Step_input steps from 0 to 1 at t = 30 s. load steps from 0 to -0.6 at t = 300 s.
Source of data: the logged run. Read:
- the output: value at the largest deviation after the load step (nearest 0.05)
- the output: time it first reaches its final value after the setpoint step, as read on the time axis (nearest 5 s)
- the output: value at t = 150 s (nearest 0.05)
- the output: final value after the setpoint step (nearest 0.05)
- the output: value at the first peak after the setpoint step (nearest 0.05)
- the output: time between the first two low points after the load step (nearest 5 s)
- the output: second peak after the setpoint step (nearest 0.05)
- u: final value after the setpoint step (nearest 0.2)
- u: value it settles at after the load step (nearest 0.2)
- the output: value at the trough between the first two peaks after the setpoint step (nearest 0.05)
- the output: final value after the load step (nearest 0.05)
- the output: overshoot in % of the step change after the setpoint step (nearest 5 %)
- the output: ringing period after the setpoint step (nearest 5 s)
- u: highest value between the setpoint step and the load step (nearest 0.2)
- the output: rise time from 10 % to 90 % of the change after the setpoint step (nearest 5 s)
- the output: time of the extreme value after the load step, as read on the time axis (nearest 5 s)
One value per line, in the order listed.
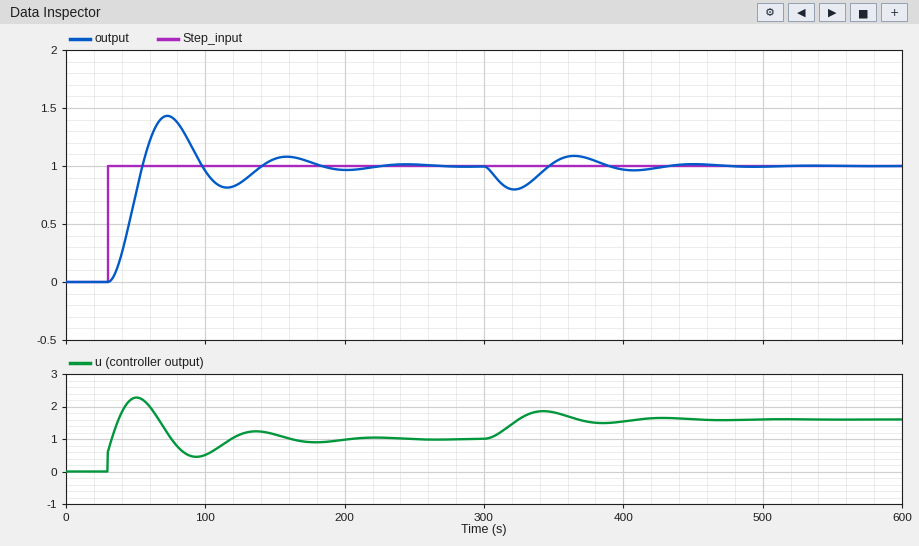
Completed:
0.80
55 s
1.05
1.00
1.45
85 s
1.10
1.0
1.6
0.80
1.00
45 %
85 s
2.2
15 s
320 s
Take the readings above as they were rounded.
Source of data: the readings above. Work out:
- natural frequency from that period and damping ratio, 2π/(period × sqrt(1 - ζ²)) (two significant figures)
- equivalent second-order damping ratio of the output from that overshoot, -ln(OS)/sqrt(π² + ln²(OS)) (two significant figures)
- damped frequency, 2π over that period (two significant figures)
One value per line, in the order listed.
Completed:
0.076 rad/s
0.25
0.074 rad/s
